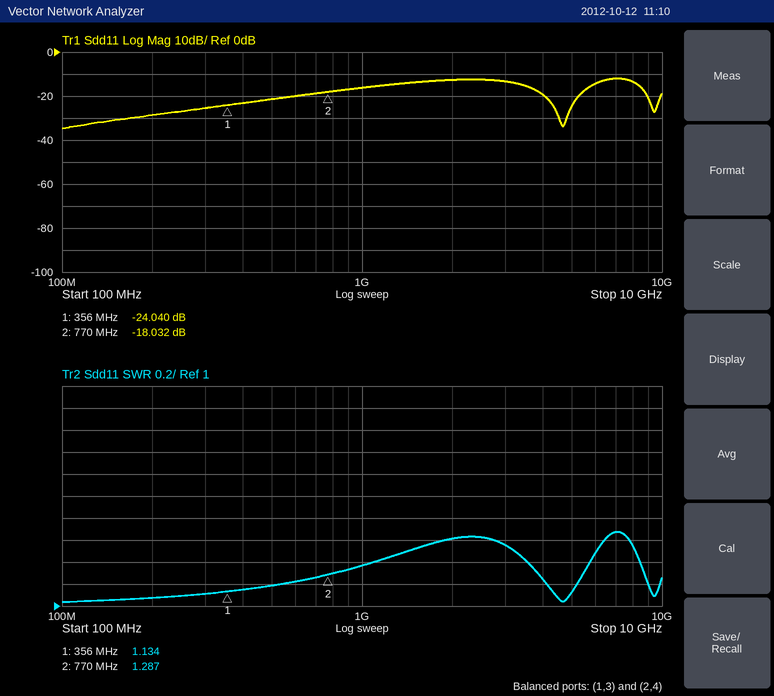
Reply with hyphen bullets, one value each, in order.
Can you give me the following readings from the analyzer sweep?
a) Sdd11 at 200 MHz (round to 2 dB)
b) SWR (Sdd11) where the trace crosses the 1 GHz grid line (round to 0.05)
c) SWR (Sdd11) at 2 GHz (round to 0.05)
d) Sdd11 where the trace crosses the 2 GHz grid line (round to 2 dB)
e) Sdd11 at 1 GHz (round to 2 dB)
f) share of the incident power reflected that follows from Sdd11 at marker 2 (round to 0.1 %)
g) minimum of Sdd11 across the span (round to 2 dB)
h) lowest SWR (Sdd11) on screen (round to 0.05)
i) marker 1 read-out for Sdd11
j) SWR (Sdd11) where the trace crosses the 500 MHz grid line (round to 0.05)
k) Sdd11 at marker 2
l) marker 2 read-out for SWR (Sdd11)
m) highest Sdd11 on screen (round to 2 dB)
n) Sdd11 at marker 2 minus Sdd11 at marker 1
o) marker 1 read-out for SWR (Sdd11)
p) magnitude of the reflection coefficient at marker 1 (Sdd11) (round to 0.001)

- -28 dB
- 1.35
- 1.60
- -12 dB
- -16 dB
- 1.6 %
- -34 dB
- 1.05
- -24.040 dB
- 1.20
- -18.032 dB
- 1.287
- -12 dB
- 6.008 dB
- 1.134
- 0.063
